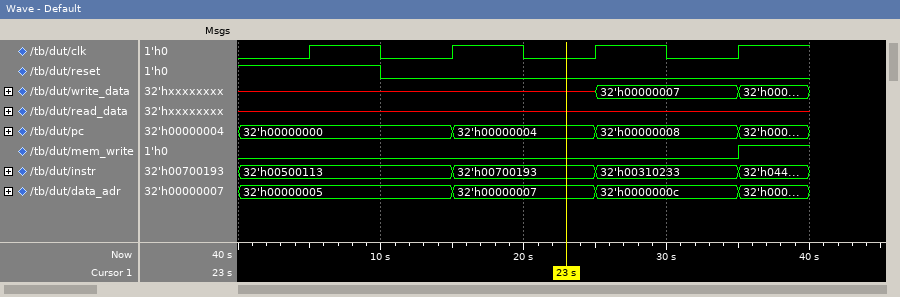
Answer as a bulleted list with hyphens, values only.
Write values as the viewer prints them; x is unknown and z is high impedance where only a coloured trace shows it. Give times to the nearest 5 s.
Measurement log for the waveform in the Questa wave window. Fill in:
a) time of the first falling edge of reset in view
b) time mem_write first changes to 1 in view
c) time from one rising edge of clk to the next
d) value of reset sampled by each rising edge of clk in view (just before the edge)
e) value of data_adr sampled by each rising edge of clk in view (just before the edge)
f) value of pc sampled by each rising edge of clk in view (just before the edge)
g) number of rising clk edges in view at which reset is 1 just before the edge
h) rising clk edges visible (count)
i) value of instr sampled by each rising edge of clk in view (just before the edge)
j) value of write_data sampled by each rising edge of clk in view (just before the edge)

- 10 s
- 35 s
- 10 s
- 1 0 0 0
- 32'h00000005, 32'h00000005, 32'h00000007, 32'h0000000c
- 32'h00000000, 32'h00000000, 32'h00000004, 32'h00000008
- 1
- 4
- 32'h00500113, 32'h00500113, 32'h00700193, 32'h00310233
- x, x, x, 32'h00000007
